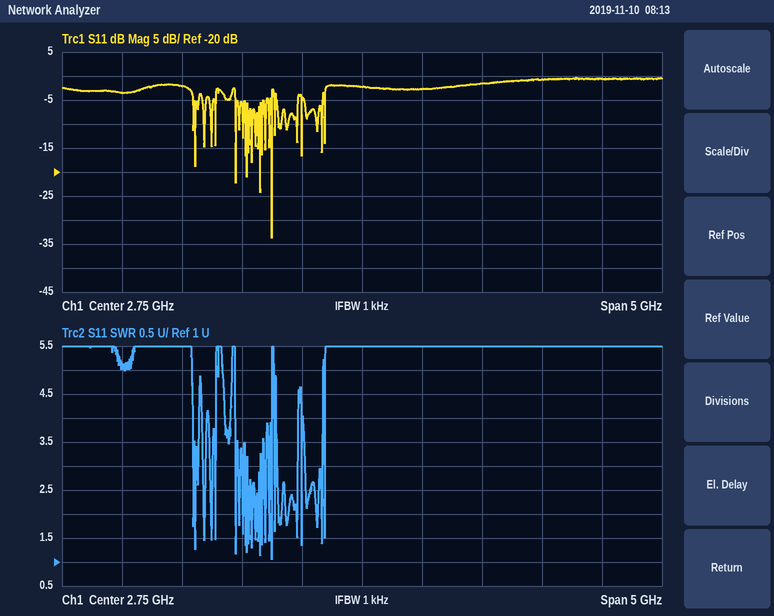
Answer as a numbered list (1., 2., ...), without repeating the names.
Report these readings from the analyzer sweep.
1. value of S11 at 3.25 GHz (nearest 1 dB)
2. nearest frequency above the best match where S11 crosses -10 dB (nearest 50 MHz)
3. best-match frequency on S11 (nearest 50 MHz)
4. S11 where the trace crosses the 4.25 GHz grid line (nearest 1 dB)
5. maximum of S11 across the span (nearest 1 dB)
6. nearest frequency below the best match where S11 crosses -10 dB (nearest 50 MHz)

1. -3 dB
2. 2.00 GHz
3. 2.00 GHz
4. -1 dB
5. 0 dB
6. 2.00 GHz
